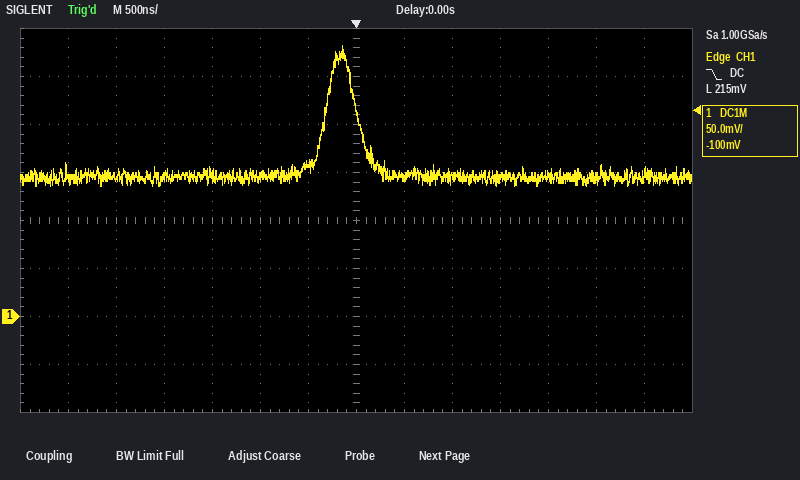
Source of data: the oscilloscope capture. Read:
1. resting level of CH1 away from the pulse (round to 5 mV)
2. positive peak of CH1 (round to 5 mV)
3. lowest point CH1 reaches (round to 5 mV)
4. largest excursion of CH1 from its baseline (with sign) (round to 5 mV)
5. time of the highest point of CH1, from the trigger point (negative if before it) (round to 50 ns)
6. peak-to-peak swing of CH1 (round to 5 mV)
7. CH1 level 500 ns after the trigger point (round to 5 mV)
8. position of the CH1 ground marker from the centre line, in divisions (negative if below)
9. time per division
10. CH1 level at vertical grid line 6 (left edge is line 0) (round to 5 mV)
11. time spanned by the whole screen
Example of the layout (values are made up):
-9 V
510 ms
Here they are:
145 mV
280 mV
135 mV
+135 mV
-150 ns
145 mV
145 mV
-2.0 div
500 ns
160 mV
7 µs
